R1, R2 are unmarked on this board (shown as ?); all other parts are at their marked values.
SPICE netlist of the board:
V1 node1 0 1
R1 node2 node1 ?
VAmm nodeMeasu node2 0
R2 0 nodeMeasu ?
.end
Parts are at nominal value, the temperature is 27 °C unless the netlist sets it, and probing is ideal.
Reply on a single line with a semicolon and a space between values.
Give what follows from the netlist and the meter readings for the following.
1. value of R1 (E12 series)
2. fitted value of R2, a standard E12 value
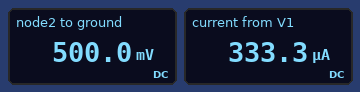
1.5 kΩ; 1.5 kΩ
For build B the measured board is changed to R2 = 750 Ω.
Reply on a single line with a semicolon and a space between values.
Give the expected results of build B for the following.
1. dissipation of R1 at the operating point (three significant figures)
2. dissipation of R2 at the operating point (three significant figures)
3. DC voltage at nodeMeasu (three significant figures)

296 µW; 148 µW; 333 mV
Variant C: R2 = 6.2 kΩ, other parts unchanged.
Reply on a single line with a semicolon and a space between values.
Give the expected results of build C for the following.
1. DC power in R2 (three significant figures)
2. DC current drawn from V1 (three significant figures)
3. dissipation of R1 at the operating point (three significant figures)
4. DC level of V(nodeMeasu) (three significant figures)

105 µW; 130 µA; 25.3 µW; 805 mV
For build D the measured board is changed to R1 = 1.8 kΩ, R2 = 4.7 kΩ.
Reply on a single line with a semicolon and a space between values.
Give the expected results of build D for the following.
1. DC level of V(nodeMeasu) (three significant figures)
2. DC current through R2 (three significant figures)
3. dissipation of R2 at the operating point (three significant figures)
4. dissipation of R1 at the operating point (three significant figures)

723 mV; 154 µA; 111 µW; 42.6 µW
